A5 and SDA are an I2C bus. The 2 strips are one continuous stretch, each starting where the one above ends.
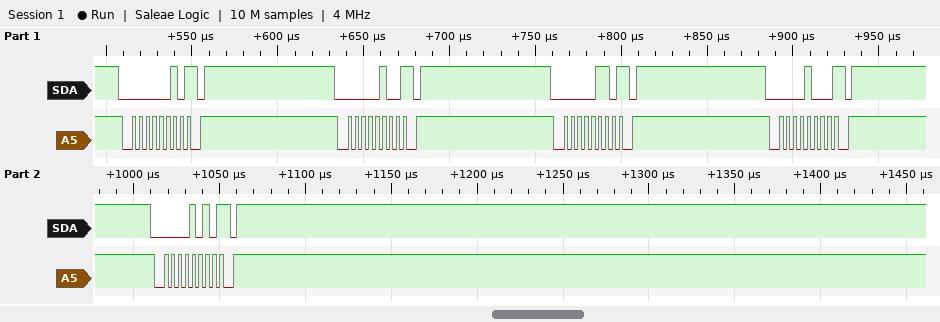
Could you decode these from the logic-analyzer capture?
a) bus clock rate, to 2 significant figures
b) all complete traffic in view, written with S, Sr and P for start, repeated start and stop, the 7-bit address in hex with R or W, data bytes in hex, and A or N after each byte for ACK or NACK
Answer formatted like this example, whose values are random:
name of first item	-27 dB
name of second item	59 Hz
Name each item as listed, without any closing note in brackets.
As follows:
bus clock rate, to 2 significant figures	250 kHz
all complete traffic in view, written with S, Sr and P for start, repeated start and stop, the 7-bit address in hex with R or W, data bytes in hex, and A or N after each byte for ACK or NACK	S 01W N P S 02W N P S 03W N P S 04W N P S 05W N P
